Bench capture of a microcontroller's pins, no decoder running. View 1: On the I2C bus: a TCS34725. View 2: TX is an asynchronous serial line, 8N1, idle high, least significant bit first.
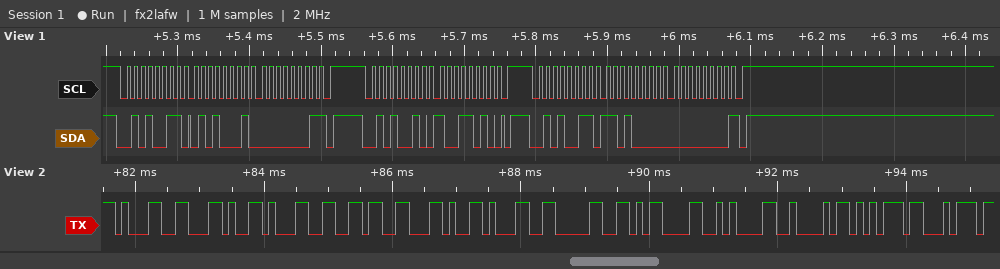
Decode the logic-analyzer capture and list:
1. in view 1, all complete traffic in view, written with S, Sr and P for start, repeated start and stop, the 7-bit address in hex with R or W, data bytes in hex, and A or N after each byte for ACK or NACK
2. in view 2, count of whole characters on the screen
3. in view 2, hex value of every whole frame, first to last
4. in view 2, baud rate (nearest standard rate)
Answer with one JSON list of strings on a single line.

["S 29R A 51 A 01 N P S 29W A 9A A P S 29R A D0 A 00 N P", "12", "31 2C 31 36 2C 31 30 0D 0A 42 75 74", "9600 baud"]
